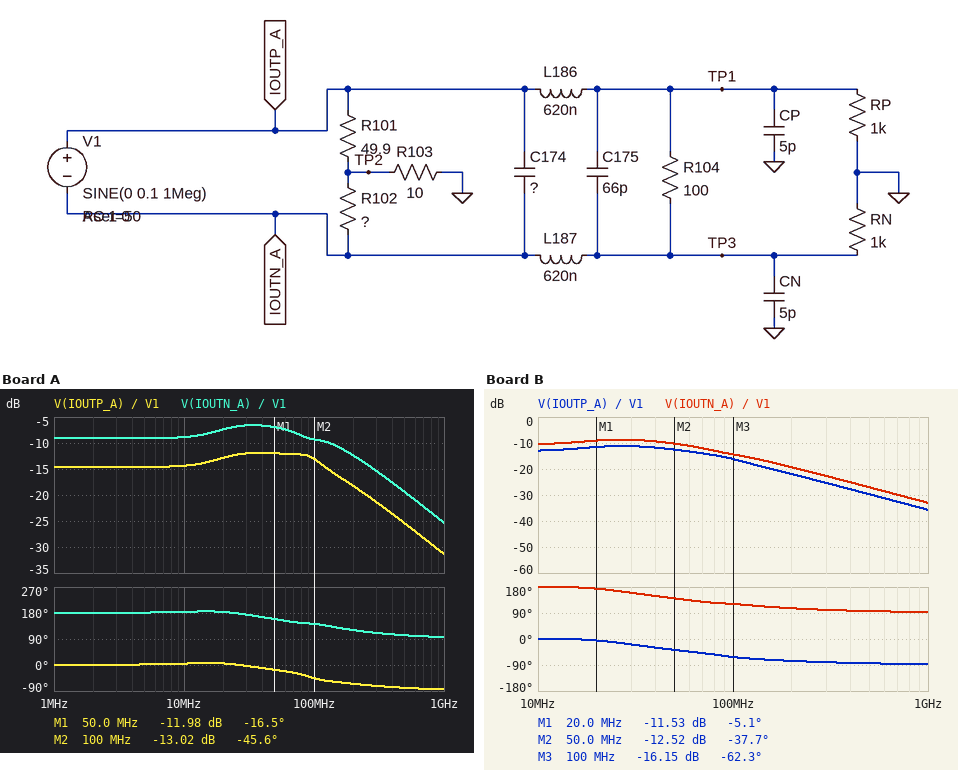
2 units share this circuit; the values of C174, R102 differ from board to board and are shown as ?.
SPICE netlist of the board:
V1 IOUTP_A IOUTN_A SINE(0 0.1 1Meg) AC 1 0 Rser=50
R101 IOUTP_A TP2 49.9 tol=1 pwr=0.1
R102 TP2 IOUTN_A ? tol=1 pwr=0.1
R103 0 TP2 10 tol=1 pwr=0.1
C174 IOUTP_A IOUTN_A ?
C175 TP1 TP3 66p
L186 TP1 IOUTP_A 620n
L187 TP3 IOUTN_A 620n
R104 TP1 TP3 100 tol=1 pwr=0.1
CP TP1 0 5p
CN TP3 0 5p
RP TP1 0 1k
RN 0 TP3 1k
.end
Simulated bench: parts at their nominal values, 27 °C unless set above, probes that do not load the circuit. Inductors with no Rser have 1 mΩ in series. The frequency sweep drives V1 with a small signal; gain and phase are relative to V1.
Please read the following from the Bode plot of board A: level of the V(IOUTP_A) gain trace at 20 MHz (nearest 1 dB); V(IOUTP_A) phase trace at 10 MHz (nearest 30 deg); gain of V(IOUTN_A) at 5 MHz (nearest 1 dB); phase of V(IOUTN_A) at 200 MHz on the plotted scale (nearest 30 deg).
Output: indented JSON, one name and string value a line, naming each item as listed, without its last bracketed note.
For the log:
{
  "level of the V(IOUTP_A) gain trace at 20 MHz": "-13 dB",
  "V(IOUTP_A) phase trace at 10 MHz": "0 deg",
  "gain of V(IOUTN_A) at 5 MHz": "-9 dB",
  "phase of V(IOUTN_A) at 200 MHz on the plotted scale": "120 deg"
}
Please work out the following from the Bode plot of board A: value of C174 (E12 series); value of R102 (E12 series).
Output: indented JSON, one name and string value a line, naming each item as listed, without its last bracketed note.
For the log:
{
  "value of C174": "39 pF",
  "value of R102": "100 Ω"
}
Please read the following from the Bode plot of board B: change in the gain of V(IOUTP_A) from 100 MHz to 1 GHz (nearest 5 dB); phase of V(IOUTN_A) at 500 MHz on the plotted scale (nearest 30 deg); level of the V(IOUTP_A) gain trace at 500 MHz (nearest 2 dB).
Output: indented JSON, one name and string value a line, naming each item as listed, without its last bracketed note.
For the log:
{
  "change in the gain of V(IOUTP_A) from 100 MHz to 1 GHz": "-20 dB",
  "phase of V(IOUTN_A) at 500 MHz on the plotted scale": "90 deg",
  "level of the V(IOUTP_A) gain trace at 500 MHz": "-30 dB"
}
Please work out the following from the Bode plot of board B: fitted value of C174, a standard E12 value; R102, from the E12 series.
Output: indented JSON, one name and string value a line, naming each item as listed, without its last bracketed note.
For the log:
{
  "fitted value of C174, a standard E12 value": "82 pF",
  "R102, from the E12 series": "68 Ω"
}
